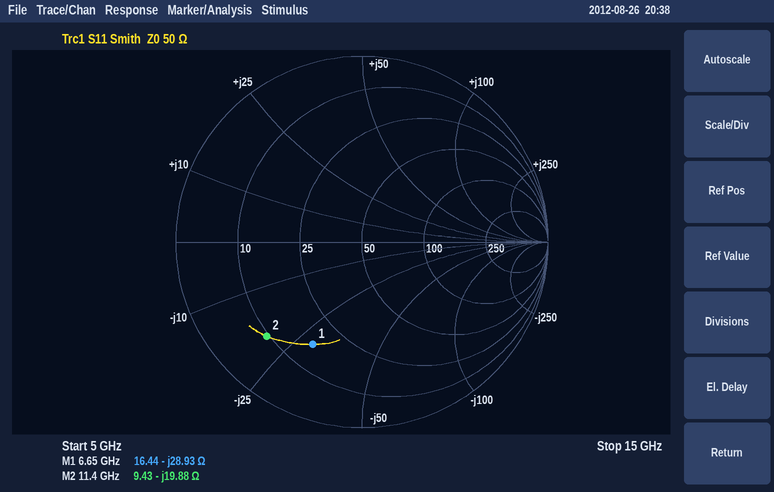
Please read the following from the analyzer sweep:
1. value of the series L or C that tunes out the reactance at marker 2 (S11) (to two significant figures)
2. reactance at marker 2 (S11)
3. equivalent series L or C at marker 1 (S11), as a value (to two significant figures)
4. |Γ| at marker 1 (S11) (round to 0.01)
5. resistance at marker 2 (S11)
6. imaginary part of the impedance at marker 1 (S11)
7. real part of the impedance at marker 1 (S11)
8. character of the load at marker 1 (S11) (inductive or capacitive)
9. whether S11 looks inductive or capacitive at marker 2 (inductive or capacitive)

280 pH
-19.88 Ω
830 fF
0.61
9.43 Ω
-28.93 Ω
16.44 Ω
capacitive
capacitive
